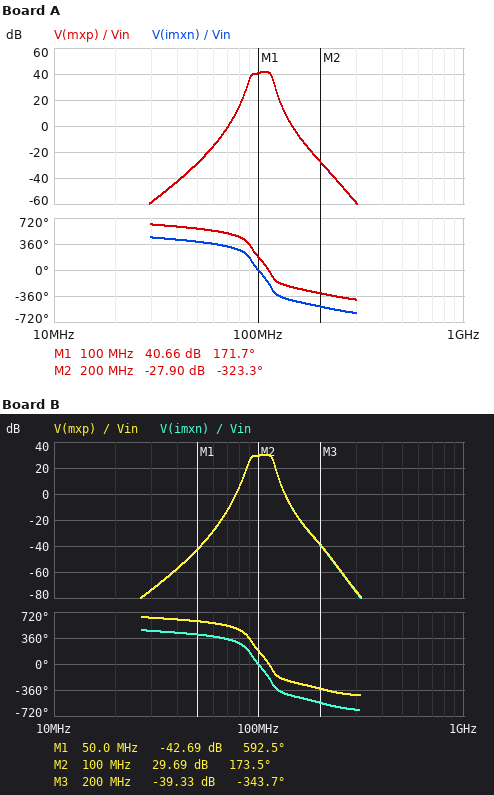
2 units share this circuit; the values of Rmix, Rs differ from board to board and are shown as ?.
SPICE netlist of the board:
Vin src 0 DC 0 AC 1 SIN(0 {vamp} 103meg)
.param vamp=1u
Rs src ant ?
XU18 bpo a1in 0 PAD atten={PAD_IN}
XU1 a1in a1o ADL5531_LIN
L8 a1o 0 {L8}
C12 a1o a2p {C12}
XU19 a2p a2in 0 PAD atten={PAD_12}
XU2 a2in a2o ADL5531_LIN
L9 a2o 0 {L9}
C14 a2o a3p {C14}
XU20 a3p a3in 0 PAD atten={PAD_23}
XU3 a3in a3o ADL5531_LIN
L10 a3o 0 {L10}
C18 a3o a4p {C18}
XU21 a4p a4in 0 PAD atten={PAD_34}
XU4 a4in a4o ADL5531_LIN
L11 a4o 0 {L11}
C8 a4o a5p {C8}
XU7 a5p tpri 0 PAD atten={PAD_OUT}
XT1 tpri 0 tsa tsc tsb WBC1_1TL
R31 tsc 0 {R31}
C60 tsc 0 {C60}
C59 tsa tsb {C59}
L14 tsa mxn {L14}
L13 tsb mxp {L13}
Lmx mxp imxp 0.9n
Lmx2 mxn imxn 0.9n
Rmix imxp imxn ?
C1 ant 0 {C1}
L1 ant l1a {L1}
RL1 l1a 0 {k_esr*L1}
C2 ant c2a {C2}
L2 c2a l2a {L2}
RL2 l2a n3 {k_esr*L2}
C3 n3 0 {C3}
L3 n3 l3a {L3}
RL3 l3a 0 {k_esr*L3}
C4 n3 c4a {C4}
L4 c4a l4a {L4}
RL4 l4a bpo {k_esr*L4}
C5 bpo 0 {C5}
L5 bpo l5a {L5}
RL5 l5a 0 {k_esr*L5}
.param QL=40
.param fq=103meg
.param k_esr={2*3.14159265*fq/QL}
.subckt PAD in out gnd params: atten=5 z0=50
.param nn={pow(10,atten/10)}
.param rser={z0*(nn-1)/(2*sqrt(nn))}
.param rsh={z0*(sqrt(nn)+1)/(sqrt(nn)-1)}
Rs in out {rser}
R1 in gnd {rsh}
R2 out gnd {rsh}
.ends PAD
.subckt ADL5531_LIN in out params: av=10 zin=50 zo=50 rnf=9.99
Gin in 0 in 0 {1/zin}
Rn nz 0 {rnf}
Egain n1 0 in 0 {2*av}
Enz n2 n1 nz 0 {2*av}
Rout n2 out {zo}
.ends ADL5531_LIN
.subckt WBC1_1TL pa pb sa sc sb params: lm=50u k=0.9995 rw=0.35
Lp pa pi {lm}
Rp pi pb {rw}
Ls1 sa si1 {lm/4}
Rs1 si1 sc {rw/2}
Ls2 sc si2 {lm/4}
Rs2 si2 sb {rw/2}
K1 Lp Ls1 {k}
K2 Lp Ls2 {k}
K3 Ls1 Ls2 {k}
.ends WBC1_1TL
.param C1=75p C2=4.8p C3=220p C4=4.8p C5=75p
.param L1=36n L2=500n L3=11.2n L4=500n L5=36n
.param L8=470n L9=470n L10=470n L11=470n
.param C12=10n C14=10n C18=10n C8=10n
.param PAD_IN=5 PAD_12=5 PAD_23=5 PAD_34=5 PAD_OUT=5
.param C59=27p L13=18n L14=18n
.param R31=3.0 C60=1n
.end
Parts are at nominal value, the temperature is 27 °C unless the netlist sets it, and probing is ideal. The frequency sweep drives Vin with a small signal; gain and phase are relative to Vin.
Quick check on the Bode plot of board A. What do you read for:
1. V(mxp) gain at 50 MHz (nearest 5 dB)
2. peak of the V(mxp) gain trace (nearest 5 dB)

-30 dB
40 dB
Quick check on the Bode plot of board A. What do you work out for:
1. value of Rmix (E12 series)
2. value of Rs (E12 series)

33 Ω
18 Ω
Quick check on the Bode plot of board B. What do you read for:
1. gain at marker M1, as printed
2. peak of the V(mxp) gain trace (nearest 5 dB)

-42.69 dB
30 dB
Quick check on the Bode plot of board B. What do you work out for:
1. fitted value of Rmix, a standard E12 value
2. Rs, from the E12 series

8.2 Ω
39 Ω
